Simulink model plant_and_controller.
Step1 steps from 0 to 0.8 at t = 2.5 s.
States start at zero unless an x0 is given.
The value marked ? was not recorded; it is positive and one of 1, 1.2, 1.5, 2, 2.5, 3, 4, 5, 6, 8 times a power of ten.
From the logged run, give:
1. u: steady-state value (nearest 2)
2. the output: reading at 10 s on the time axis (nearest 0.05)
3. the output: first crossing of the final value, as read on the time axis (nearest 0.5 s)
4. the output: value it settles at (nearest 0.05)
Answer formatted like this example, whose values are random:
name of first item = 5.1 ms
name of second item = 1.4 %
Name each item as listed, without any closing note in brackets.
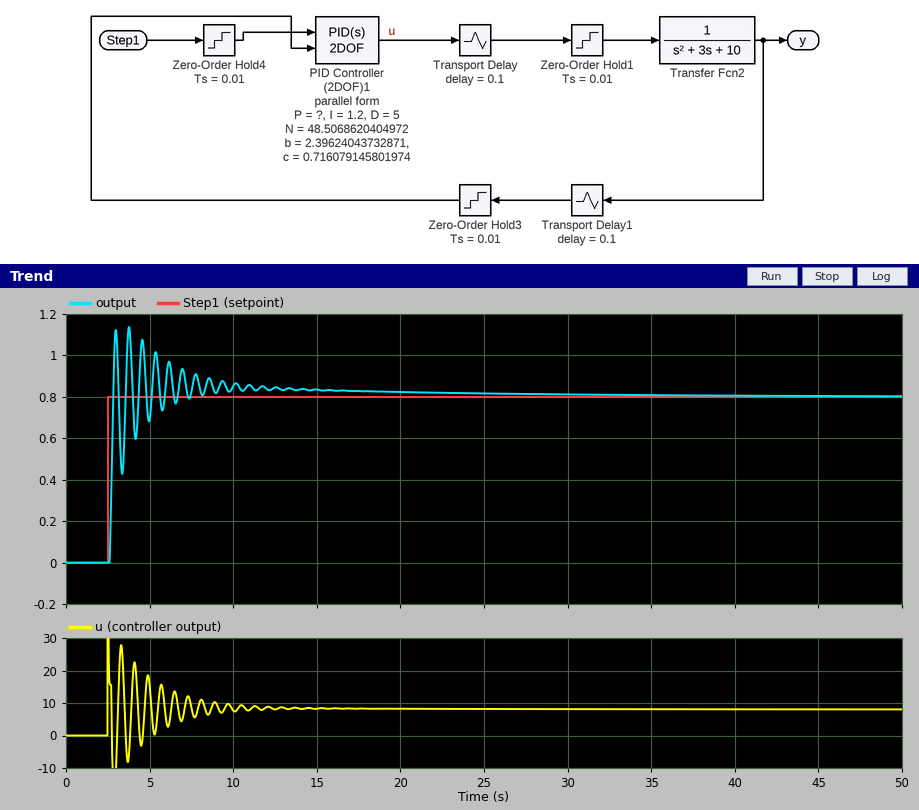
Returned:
u: steady-state value = 8
the output: reading at 10 s on the time axis = 0.85
the output: first crossing of the final value, as read on the time axis = 3.0 s
the output: value it settles at = 0.80
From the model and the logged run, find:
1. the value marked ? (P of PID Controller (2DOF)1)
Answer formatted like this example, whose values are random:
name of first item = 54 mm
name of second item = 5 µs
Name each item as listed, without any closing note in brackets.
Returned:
the value marked ? (P of PID Controller (2DOF)1) = 8
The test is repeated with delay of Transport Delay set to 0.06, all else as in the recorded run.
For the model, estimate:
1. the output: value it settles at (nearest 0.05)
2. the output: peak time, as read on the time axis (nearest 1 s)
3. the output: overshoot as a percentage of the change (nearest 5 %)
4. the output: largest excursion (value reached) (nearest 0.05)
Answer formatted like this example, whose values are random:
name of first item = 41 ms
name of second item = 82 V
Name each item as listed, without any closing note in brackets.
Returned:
the output: value it settles at = 0.80
the output: peak time, as read on the time axis = 3 s
the output: overshoot as a percentage of the change = 25 %
the output: largest excursion (value reached) = 1.00
